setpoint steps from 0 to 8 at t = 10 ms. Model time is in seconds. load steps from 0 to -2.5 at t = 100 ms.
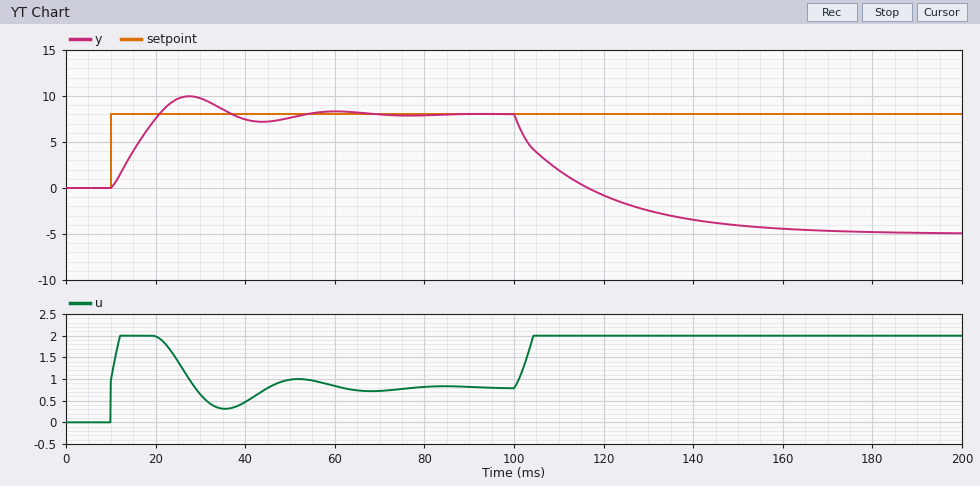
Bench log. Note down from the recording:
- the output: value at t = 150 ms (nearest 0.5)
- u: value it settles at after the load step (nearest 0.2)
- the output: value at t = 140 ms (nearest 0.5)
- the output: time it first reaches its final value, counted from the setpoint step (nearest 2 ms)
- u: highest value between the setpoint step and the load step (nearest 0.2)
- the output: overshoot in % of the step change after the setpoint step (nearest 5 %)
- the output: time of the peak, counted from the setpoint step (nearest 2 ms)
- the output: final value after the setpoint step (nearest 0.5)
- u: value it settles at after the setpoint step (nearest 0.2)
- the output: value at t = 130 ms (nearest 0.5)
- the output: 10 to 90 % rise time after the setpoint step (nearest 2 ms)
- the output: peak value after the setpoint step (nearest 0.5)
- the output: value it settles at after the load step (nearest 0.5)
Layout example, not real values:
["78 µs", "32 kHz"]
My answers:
["-4.0", "2.0", "-3.5", "10 ms", "2.0", "25 %", "18 ms", "8.0", "0.8", "-2.5", "8 ms", "10.0", "-5.0"]
